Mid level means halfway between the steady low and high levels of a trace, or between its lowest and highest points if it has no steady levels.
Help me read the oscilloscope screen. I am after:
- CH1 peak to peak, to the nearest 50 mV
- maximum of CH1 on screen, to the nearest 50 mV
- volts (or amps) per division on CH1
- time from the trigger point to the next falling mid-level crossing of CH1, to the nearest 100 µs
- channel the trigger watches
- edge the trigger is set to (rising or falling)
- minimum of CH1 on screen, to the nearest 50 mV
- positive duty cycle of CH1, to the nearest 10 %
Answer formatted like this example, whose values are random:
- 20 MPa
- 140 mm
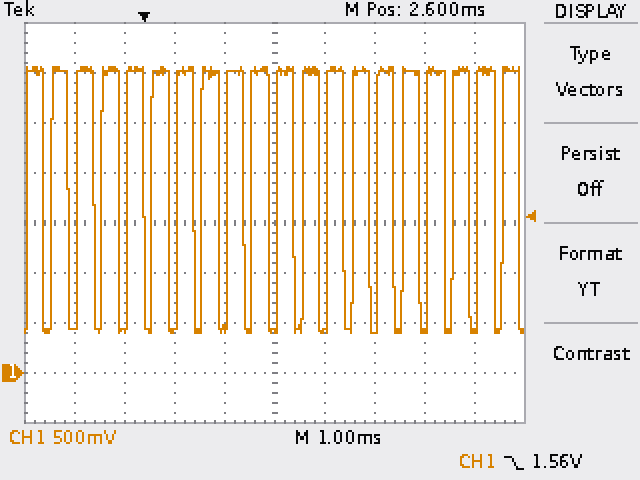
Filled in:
- 2.65 V
- 3.05 V
- 500 mV
- 500 µs
- CH1
- falling
- 400 mV
- 70 %
